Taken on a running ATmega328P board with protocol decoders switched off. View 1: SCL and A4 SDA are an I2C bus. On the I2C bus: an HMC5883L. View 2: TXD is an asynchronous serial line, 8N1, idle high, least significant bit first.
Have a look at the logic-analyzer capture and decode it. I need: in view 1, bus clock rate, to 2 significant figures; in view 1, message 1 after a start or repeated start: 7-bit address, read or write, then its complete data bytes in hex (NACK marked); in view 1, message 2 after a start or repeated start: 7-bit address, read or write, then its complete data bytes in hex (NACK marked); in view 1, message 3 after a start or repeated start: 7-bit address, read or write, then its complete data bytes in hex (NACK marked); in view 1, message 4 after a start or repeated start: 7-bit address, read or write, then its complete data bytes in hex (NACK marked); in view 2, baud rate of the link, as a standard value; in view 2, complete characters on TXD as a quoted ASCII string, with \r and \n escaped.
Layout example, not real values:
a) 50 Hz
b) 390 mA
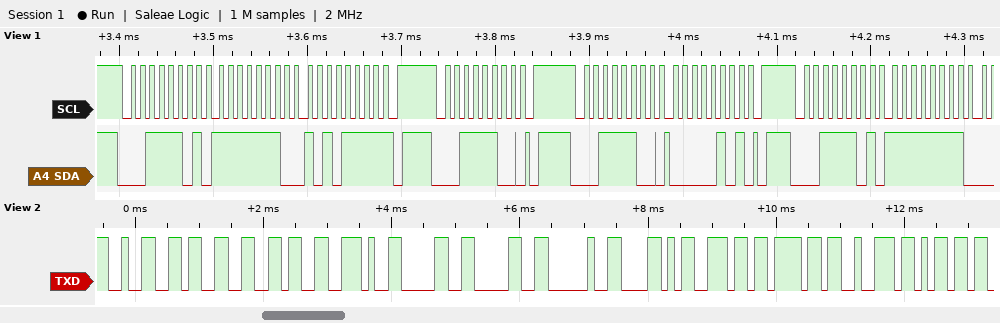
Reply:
a) 100 kHz
b) 0x1E read: FE AF NACK
c) 0x1E write
d) 0x1E write: 05
e) 0x1E read: FF
f) 9600 baud
g) "236.00 Xnorm"
